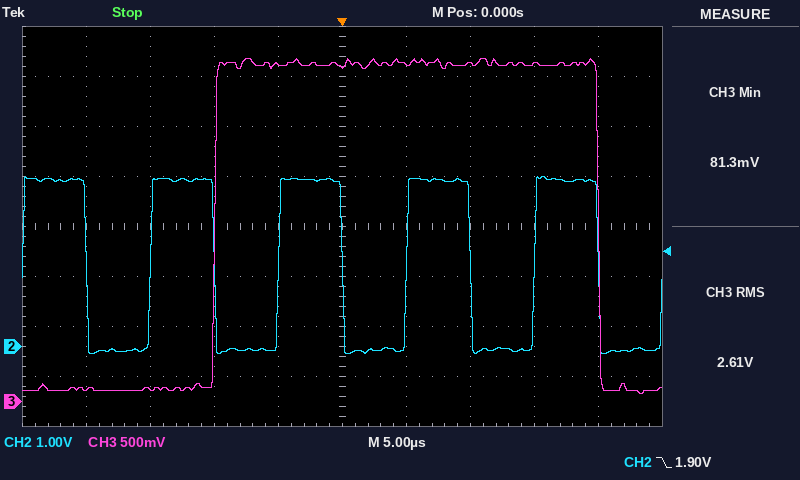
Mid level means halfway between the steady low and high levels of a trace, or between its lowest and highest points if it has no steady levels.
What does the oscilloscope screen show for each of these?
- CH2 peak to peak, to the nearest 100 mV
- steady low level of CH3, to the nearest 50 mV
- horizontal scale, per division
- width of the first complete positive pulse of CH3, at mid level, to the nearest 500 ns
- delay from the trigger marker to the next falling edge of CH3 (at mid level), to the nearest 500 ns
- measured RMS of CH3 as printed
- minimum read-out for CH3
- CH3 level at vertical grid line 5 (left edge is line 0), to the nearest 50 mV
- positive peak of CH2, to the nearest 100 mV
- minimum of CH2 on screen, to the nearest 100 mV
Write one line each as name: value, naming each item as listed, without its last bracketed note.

CH2 peak to peak, to the nearest 100 mV: 3.5 V
steady low level of CH3, to the nearest 50 mV: 100 mV
horizontal scale, per division: 5 µs
width of the first complete positive pulse of CH3, at mid level, to the nearest 500 ns: 30.0 µs
delay from the trigger marker to the next falling edge of CH3 (at mid level), to the nearest 500 ns: 20.0 µs
measured RMS of CH3 as printed: 2.61 V
minimum read-out for CH3: 81.3 mV
CH3 level at vertical grid line 5 (left edge is line 0), to the nearest 50 mV: 3.35 V
positive peak of CH2, to the nearest 100 mV: 3.4 V
minimum of CH2 on screen, to the nearest 100 mV: -100 mV
